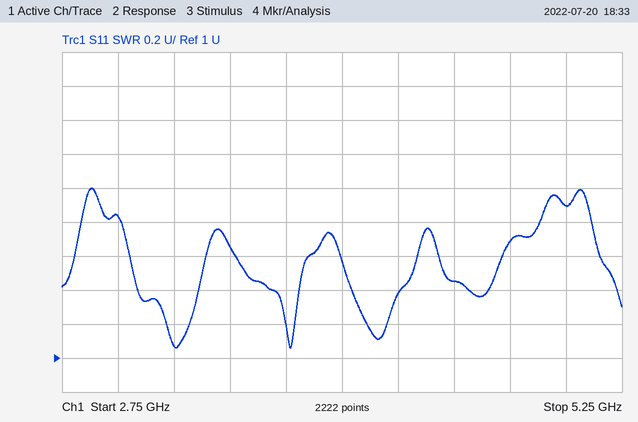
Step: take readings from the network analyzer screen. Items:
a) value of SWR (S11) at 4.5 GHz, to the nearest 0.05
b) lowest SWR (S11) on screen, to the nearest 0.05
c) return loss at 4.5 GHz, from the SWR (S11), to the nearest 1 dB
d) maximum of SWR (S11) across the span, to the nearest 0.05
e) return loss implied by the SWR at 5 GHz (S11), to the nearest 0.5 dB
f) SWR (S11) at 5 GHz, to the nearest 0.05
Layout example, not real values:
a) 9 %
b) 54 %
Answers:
a) 1.45
b) 1.05
c) 15 dB
d) 2.00
e) 10.0 dB
f) 1.90
